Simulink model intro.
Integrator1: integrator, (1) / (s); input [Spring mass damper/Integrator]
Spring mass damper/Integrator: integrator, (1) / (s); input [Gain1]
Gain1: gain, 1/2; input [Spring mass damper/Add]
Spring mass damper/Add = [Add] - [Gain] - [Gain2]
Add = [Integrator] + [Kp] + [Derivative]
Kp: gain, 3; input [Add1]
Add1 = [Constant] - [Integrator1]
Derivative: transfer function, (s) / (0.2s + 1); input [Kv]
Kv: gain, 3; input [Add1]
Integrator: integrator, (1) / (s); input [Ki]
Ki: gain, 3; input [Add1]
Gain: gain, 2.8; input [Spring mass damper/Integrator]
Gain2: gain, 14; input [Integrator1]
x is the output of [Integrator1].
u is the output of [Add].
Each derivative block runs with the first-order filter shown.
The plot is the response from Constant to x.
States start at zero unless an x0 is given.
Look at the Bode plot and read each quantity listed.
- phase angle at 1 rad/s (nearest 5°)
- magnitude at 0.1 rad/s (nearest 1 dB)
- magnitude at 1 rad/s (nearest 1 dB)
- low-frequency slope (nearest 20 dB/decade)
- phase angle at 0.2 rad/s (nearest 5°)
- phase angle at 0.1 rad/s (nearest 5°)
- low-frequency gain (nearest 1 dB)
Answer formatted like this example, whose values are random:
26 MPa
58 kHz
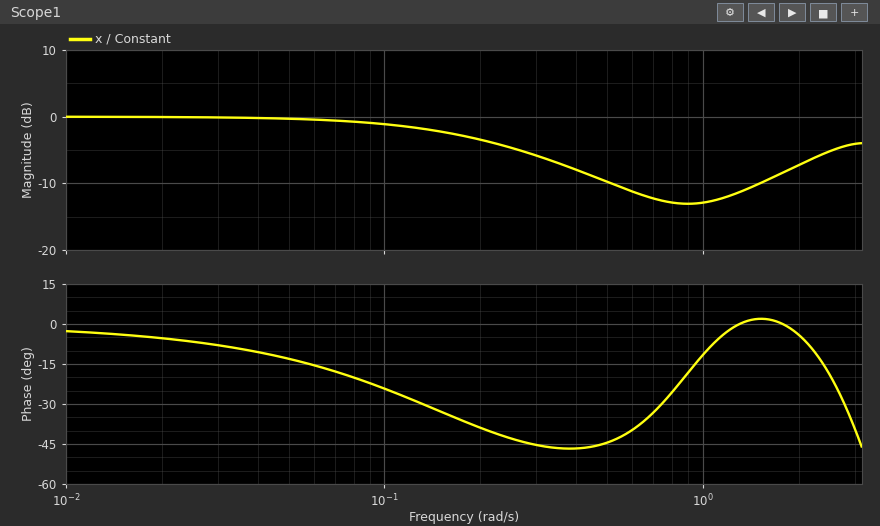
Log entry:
-10°
-1 dB
-13 dB
0 dB/decade
-40°
-25°
0 dB
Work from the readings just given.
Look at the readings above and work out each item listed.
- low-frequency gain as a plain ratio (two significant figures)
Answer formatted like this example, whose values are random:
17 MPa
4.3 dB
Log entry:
1.0
